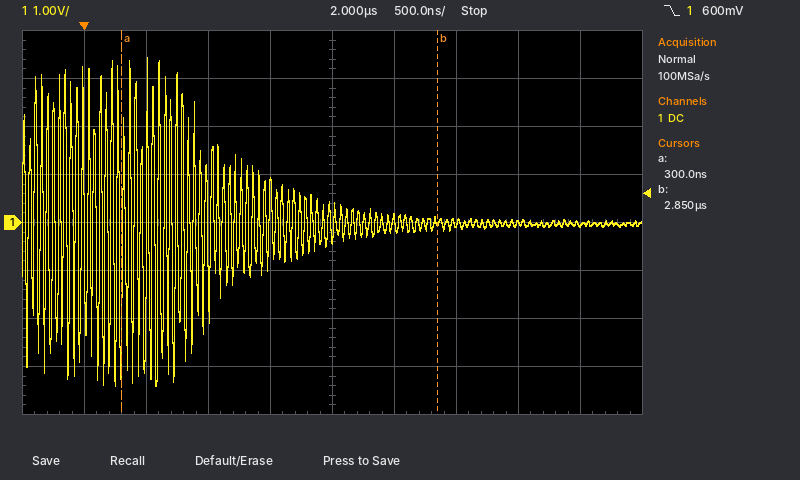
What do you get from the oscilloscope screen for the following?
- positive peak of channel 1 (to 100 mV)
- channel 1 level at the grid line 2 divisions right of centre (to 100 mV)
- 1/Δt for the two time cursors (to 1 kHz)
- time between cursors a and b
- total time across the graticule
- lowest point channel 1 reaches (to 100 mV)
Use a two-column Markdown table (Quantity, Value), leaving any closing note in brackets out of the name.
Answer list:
| Quantity | Value |
|---|---|
| positive peak of channel 1 | 3.4 V |
| channel 1 level at the grid line 2 divisions right of centre | 0.0 V |
| 1/Δt for the two time cursors | 392 kHz |
| time between cursors a and b | 2.55 µs |
| total time across the graticule | 5 µs |
| lowest point channel 1 reaches | -3.4 V |
